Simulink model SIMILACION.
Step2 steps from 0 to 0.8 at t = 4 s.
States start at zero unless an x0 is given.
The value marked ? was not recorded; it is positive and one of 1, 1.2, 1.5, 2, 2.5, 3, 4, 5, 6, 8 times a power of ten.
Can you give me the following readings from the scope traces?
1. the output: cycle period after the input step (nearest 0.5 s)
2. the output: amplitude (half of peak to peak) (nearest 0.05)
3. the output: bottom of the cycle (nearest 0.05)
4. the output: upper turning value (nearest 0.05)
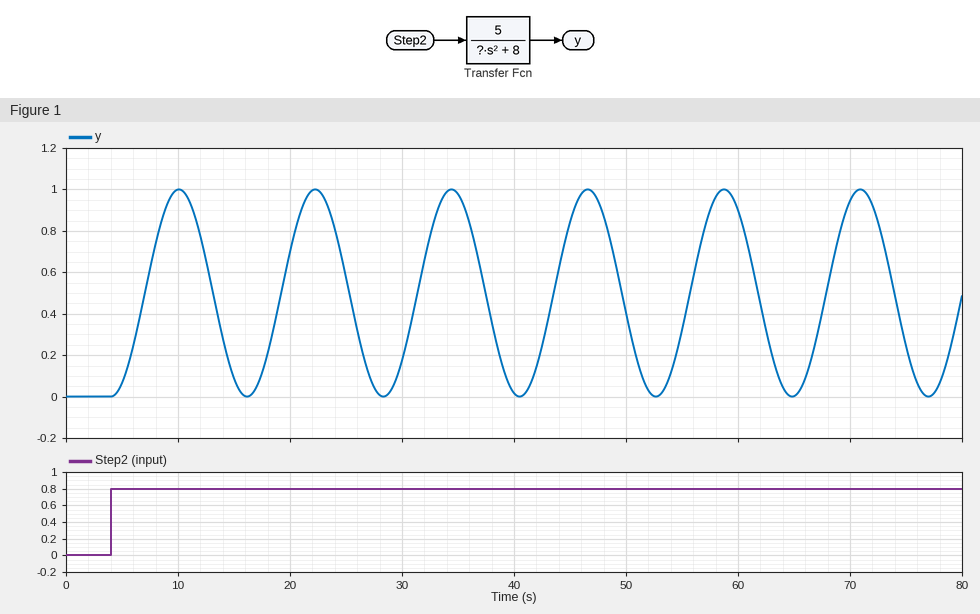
12.0 s
0.50
0.00
1.00
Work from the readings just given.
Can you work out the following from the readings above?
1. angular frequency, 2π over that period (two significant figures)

0.52 rad/s
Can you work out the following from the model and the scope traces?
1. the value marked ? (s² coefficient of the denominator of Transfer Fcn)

30
